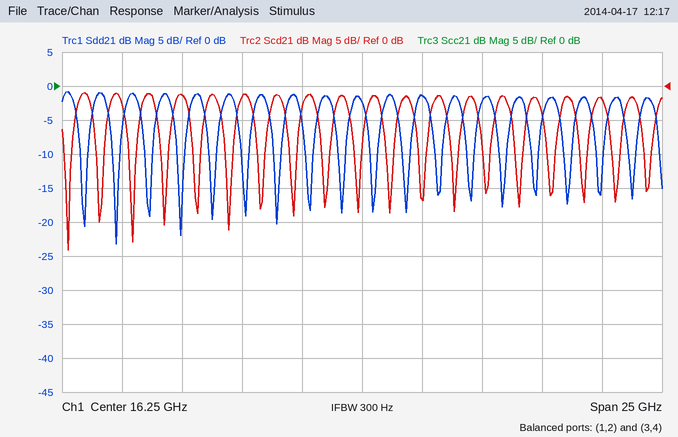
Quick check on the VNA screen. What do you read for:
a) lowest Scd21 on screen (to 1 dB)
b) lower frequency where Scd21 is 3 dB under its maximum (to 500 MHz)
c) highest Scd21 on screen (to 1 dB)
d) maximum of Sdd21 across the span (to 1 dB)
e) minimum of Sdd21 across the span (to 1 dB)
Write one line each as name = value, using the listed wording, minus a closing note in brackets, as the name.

lowest Scd21 on screen = -24 dB
lower frequency where Scd21 is 3 dB under its maximum = 4.5 GHz
highest Scd21 on screen = -1 dB
maximum of Sdd21 across the span = -1 dB
minimum of Sdd21 across the span = -23 dB
